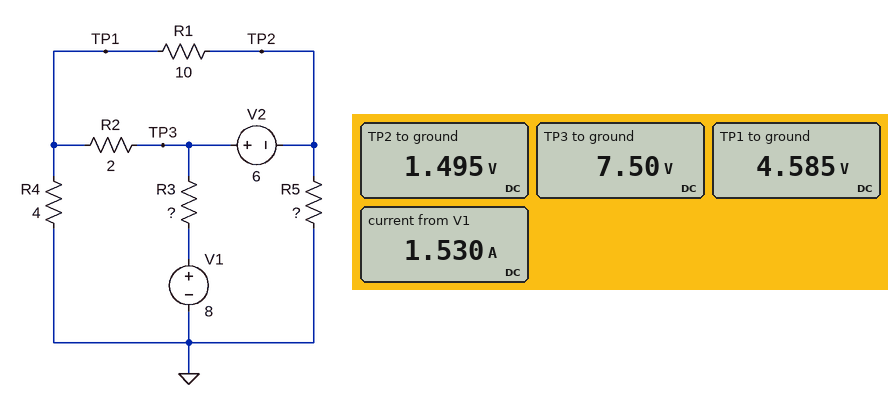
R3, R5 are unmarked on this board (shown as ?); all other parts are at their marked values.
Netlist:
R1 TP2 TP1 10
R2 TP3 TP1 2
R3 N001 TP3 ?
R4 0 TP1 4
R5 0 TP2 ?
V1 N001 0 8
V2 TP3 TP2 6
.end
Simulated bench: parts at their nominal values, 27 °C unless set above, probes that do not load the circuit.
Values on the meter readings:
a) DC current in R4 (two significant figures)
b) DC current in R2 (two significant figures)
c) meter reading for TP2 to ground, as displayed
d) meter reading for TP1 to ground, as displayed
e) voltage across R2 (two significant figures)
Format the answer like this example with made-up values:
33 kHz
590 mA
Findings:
1.1 A
1.5 A
1.495 V
4.585 V
2.9 V
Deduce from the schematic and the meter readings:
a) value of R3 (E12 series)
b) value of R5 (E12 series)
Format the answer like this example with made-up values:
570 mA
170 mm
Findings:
0.33 Ω
3.9 Ω
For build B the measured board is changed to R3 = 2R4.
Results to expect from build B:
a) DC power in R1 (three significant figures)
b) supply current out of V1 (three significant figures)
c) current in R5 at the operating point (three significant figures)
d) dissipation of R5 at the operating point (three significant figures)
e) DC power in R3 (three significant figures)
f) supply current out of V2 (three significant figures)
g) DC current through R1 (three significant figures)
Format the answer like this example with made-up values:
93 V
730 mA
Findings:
1.26 W
857 mA
14.8 mA
854 µW
1.76 W
369 mA
355 mA
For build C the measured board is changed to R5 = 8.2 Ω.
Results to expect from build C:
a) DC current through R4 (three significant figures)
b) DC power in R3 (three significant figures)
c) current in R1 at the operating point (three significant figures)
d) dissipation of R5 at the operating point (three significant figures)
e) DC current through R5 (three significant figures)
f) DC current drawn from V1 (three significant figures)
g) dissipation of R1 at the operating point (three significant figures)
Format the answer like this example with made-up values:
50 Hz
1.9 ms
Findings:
1.16 A
598 mW
307 mA
295 mW
190 mA
1.35 A
944 mW
